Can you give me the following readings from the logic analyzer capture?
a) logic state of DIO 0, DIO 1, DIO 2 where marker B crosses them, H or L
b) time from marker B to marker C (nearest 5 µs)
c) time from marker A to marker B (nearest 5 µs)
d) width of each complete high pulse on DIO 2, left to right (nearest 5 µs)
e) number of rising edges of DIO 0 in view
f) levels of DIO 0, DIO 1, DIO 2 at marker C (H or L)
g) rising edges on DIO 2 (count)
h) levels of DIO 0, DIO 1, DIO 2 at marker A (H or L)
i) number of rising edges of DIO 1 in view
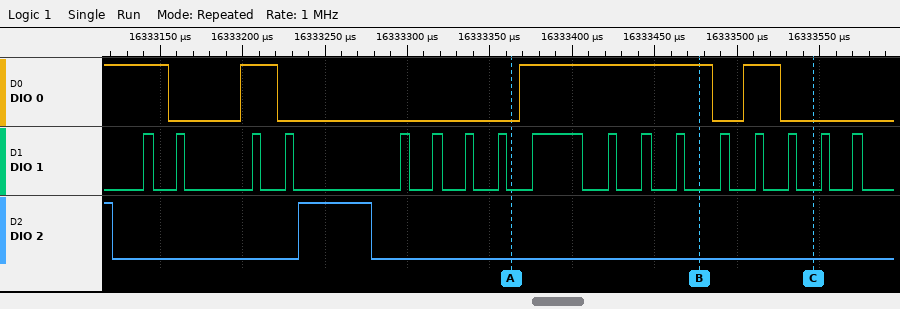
DIO 0=H, DIO 1=L, DIO 2=L
70 µs
115 µs
45 µs
3
DIO 0=L, DIO 1=L, DIO 2=L
1
DIO 0=L, DIO 1=L, DIO 2=L
17
